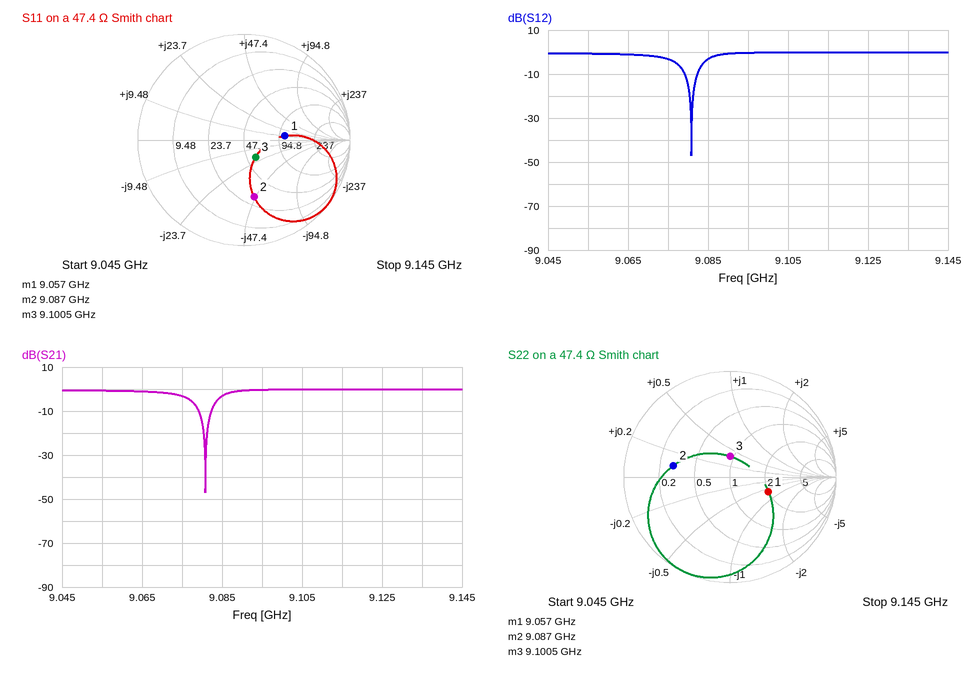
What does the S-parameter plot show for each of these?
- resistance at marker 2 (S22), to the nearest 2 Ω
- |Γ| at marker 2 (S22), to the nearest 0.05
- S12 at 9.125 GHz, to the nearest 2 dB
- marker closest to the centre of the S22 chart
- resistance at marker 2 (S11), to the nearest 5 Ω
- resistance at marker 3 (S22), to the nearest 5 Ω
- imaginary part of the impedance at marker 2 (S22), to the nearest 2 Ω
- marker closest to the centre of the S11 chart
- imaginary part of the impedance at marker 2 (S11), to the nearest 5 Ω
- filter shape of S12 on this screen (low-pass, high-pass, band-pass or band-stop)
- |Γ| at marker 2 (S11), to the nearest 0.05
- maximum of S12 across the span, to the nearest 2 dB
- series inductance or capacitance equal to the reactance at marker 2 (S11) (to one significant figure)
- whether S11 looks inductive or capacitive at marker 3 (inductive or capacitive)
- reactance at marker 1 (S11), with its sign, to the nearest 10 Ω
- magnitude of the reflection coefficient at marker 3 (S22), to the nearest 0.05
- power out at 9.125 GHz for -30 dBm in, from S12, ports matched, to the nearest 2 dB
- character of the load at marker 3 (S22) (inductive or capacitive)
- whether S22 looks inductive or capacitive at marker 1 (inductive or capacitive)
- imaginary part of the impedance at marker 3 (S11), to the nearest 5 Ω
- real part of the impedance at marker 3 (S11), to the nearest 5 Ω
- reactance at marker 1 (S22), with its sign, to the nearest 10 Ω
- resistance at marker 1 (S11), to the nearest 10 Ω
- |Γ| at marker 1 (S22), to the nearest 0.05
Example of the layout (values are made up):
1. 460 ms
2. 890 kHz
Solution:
1. 14 Ω
2. 0.55
3. 0 dB
4. marker 3
5. 30 Ω
6. 45 Ω
7. +4 Ω
8. marker 3
9. -45 Ω
10. band-stop
11. 0.55
12. 0 dB
13. 400 fF
14. capacitive
15. +10 Ω
16. 0.20
17. -30 dBm
18. inductive
19. capacitive
20. -20 Ω
21. 55 Ω
22. -30 Ω
23. 110 Ω
24. 0.40
